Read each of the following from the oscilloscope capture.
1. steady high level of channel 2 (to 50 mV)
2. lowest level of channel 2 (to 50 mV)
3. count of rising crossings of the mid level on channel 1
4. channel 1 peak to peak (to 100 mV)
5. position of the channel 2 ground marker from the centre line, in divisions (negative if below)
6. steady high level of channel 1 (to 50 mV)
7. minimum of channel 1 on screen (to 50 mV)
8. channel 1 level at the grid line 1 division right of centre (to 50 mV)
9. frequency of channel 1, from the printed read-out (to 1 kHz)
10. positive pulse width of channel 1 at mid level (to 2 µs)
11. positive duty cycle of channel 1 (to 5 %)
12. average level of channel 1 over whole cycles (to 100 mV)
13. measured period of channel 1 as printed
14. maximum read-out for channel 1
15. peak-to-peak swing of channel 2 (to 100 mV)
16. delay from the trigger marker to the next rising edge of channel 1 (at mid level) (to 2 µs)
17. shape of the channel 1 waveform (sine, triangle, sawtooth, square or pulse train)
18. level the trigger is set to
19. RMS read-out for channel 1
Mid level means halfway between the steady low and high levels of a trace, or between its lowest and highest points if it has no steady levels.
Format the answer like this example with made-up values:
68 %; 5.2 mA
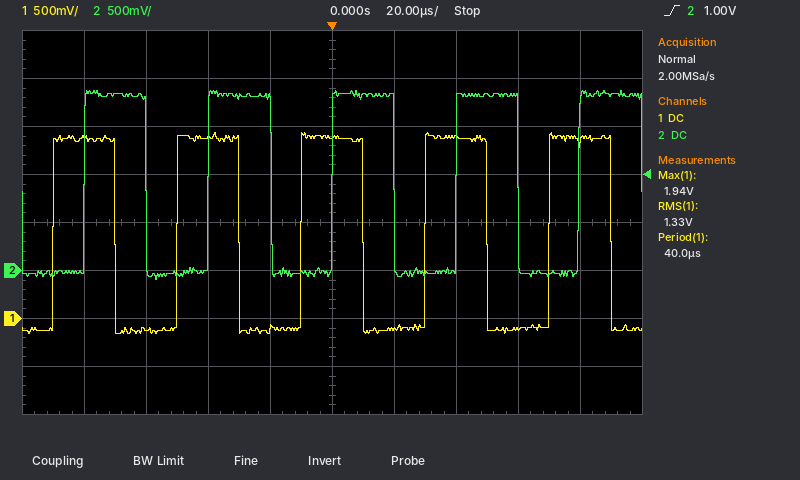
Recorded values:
1.85 V; -100 mV; 5; 2.10 V; -1.0 div; 1.90 V; -150 mV; -100 mV; 25 kHz; 20 µs; 50 %; 900 mV; 40.0 µs; 1.94 V; 2.00 V; 30 µs; square; 1.00 V; 1.33 V
